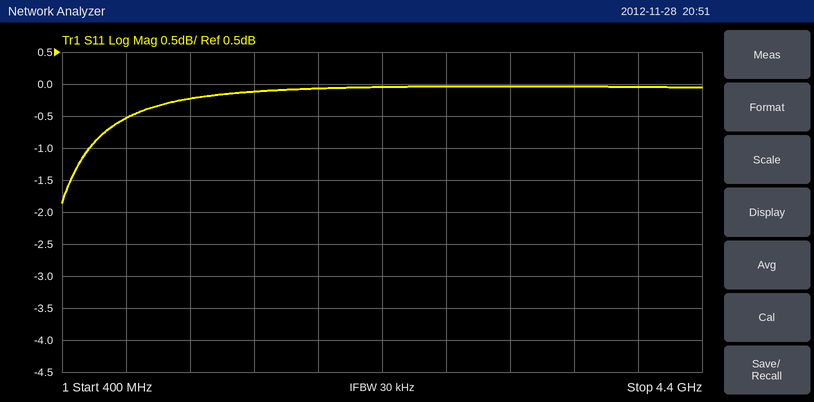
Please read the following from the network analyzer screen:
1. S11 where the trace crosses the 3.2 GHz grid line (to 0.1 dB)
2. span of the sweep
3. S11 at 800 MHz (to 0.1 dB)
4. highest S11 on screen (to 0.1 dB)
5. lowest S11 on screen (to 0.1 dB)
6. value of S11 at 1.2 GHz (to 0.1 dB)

0.0 dB
4 GHz
-0.5 dB
0.0 dB
-1.9 dB
-0.2 dB
